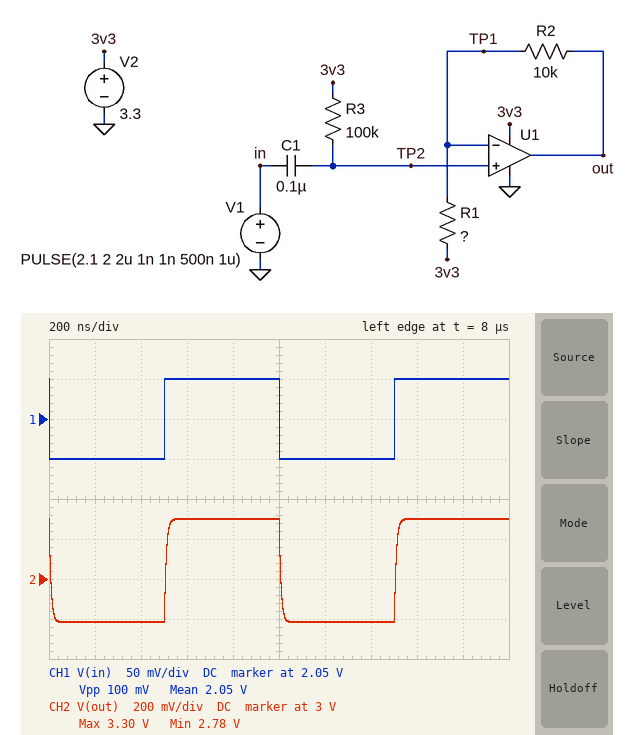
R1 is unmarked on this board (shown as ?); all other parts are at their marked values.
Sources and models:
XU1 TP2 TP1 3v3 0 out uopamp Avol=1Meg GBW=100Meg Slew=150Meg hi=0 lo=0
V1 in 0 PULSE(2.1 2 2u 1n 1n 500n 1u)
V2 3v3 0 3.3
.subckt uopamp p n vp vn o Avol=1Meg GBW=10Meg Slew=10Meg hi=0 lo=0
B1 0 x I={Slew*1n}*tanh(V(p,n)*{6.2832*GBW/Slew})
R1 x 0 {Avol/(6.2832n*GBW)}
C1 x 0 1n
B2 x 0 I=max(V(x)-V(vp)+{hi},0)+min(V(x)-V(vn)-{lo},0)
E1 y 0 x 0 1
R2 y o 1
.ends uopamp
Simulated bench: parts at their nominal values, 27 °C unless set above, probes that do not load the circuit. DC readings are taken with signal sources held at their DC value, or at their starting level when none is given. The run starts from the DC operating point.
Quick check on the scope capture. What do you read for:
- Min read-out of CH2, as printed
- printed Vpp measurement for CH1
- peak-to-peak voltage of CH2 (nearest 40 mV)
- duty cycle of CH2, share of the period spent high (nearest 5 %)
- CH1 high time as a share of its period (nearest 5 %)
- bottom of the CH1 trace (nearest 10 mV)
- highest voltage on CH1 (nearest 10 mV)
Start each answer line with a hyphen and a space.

- 2.78 V
- 100 mV
- 520 mV
- 50 %
- 50 %
- 2.00 V
- 2.10 V
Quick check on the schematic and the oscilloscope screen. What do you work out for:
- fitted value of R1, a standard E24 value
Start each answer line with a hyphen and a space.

- 2.4 kΩ
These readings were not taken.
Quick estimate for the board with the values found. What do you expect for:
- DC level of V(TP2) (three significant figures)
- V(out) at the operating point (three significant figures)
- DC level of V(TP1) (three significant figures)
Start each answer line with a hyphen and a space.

- 3.30 V
- 3.30 V
- 3.30 V
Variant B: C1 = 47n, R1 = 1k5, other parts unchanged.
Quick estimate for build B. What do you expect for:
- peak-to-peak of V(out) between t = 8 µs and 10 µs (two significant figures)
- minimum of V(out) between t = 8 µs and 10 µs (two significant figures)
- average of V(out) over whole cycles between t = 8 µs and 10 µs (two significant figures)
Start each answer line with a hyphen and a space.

- 770 mV
- 2.5 V
- 2.9 V
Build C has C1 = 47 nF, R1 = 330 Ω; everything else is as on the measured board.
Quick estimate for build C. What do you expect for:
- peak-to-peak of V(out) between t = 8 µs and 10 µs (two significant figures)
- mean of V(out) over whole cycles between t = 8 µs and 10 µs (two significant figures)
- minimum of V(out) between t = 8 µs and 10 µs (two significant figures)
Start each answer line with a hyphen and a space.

- 3.1 V
- 1.7 V
- 170 mV
